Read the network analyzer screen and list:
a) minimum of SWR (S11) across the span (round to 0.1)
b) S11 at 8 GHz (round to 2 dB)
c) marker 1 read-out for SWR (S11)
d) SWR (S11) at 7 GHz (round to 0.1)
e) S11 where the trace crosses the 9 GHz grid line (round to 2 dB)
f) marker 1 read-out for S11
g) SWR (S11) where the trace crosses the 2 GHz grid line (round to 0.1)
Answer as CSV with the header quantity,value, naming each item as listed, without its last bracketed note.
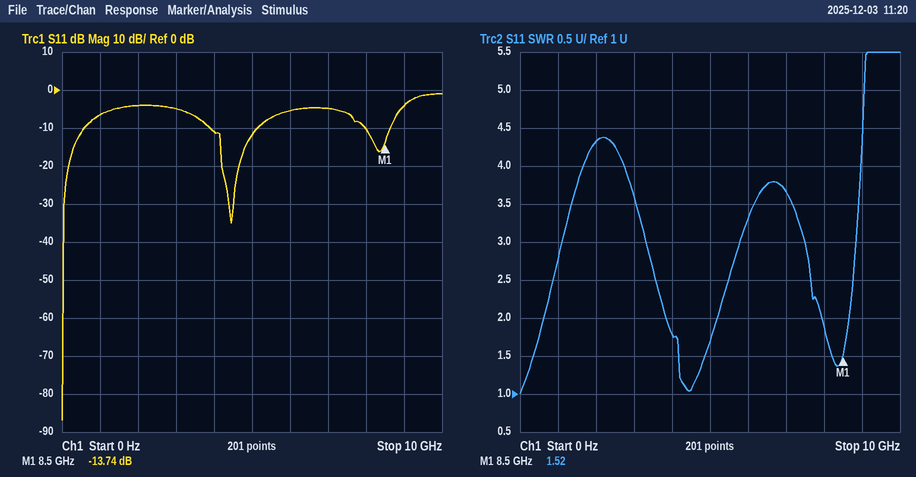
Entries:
quantity,value
minimum of SWR (S11) across the span,1.0
S11 at 8 GHz,-10 dB
marker 1 read-out for SWR,1.52
SWR (S11) at 7 GHz,3.7
S11 where the trace crosses the 9 GHz grid line,-4 dB
marker 1 read-out for S11,-13.74 dB
SWR (S11) where the trace crosses the 2 GHz grid line,4.3
